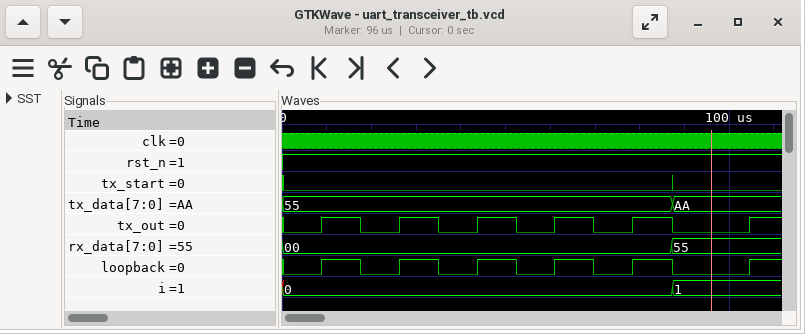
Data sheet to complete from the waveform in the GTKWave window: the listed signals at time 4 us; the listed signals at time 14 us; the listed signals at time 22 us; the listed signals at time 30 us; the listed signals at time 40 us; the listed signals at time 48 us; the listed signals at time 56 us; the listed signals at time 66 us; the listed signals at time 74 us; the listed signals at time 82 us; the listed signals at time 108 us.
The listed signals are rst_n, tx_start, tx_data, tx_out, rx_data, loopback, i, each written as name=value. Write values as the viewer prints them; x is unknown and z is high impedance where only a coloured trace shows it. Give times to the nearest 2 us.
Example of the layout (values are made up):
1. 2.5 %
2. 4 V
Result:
1. rst_n=1, tx_start=0, tx_data=55, tx_out=0, rx_data=00, loopback=0, i=0
2. rst_n=1, tx_start=0, tx_data=55, tx_out=1, rx_data=00, loopback=1, i=0
3. rst_n=1, tx_start=0, tx_data=55, tx_out=0, rx_data=00, loopback=0, i=0
4. rst_n=1, tx_start=0, tx_data=55, tx_out=1, rx_data=00, loopback=1, i=0
5. rst_n=1, tx_start=0, tx_data=55, tx_out=0, rx_data=00, loopback=0, i=0
6. rst_n=1, tx_start=0, tx_data=55, tx_out=1, rx_data=00, loopback=1, i=0
7. rst_n=1, tx_start=0, tx_data=55, tx_out=0, rx_data=00, loopback=0, i=0
8. rst_n=1, tx_start=0, tx_data=55, tx_out=1, rx_data=00, loopback=1, i=0
9. rst_n=1, tx_start=0, tx_data=55, tx_out=0, rx_data=00, loopback=0, i=0
10. rst_n=1, tx_start=0, tx_data=55, tx_out=1, rx_data=00, loopback=1, i=0
11. rst_n=1, tx_start=0, tx_data=AA, tx_out=1, rx_data=55, loopback=1, i=1
